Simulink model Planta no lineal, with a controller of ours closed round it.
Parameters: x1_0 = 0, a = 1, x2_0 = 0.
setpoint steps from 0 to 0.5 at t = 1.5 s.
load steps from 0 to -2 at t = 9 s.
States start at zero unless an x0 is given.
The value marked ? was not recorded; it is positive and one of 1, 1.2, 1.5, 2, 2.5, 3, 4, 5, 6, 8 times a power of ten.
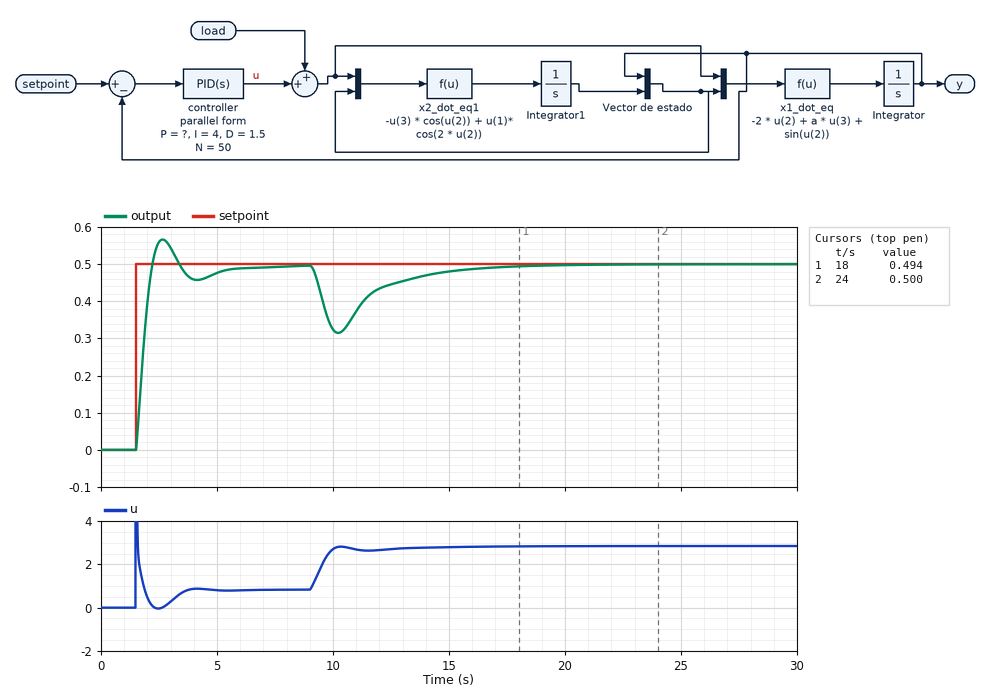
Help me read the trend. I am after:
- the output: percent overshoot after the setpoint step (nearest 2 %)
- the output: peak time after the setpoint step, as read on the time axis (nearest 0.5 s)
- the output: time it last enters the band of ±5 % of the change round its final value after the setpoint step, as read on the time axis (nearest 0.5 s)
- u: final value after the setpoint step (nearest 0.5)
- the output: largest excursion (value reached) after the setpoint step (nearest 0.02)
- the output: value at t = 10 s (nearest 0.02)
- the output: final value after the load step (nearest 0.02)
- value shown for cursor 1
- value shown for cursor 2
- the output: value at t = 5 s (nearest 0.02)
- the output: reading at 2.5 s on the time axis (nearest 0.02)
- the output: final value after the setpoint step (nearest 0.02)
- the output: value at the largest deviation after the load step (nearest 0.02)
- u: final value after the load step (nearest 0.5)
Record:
14 %
2.5 s
5.0 s
1.0
0.56
0.32
0.50
0.494
0.500
0.48
0.56
0.50
0.32
3.0
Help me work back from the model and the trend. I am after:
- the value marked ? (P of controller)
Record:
8
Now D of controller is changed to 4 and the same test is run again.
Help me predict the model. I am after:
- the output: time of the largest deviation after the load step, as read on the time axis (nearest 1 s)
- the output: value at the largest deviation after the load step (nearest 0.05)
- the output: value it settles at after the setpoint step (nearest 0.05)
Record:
10 s
0.35
0.50
